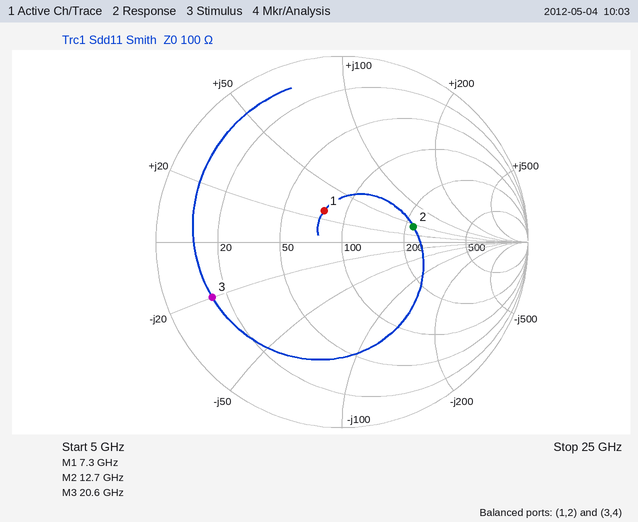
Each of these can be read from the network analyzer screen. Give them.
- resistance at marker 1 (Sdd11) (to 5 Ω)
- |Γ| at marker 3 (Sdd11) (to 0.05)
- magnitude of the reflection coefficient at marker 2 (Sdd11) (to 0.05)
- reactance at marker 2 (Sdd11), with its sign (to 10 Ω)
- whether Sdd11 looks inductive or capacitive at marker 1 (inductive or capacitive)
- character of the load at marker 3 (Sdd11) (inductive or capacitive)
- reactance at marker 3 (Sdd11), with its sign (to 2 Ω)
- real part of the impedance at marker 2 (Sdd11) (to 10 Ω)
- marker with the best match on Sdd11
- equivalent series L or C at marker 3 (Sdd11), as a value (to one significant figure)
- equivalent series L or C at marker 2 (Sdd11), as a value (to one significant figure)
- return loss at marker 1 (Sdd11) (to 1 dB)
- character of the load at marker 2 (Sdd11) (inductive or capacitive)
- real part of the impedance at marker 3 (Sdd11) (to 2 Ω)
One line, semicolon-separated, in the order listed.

80 Ω; 0.75; 0.40; +40 Ω; inductive; capacitive; -20 Ω; 220 Ω; marker 1; 400 fF; 500 pH; 14 dB; inductive; 14 Ω
